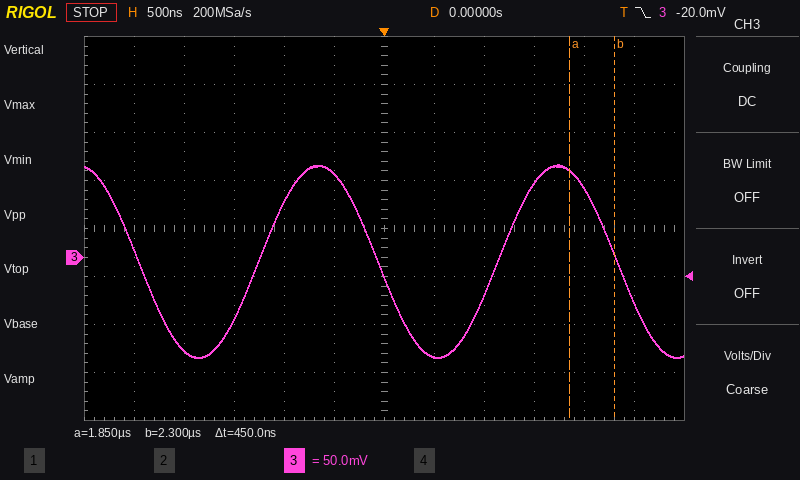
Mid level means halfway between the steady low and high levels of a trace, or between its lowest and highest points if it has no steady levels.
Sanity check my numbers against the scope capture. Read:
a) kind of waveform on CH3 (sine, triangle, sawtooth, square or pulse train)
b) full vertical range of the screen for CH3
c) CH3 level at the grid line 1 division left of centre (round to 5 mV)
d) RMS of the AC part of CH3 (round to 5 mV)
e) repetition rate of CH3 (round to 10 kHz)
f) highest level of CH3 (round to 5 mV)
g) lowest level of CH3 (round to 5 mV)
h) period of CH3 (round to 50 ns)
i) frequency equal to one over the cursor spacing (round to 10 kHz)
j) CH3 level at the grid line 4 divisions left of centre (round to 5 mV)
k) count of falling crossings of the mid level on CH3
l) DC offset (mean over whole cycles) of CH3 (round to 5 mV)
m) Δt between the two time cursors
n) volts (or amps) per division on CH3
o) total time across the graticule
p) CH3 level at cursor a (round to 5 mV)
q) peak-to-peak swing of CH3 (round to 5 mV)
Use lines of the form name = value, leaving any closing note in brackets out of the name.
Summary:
kind of waveform on CH3 = sine
full vertical range of the screen for CH3 = 400 mV
CH3 level at the grid line 1 division left of centre = 85 mV
RMS of the AC part of CH3 = 70 mV
repetition rate of CH3 = 420 kHz
highest level of CH3 = 95 mV
lowest level of CH3 = -105 mV
period of CH3 = 2.40 µs
frequency equal to one over the cursor spacing = 2.22 MHz
CH3 level at the grid line 4 divisions left of centre = -95 mV
count of falling crossings of the mid level on CH3 = 3
DC offset (mean over whole cycles) of CH3 = -5 mV
Δt between the two time cursors = 450 ns
volts (or amps) per division on CH3 = 50 mV
total time across the graticule = 6 µs
CH3 level at cursor a = 90 mV
peak-to-peak swing of CH3 = 200 mV
